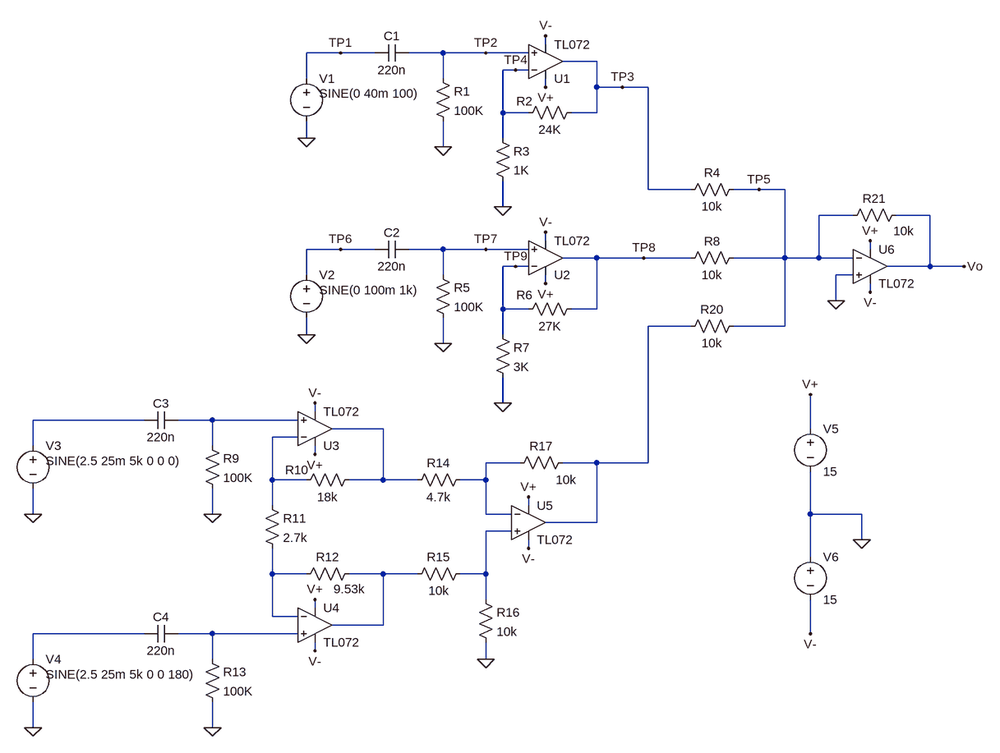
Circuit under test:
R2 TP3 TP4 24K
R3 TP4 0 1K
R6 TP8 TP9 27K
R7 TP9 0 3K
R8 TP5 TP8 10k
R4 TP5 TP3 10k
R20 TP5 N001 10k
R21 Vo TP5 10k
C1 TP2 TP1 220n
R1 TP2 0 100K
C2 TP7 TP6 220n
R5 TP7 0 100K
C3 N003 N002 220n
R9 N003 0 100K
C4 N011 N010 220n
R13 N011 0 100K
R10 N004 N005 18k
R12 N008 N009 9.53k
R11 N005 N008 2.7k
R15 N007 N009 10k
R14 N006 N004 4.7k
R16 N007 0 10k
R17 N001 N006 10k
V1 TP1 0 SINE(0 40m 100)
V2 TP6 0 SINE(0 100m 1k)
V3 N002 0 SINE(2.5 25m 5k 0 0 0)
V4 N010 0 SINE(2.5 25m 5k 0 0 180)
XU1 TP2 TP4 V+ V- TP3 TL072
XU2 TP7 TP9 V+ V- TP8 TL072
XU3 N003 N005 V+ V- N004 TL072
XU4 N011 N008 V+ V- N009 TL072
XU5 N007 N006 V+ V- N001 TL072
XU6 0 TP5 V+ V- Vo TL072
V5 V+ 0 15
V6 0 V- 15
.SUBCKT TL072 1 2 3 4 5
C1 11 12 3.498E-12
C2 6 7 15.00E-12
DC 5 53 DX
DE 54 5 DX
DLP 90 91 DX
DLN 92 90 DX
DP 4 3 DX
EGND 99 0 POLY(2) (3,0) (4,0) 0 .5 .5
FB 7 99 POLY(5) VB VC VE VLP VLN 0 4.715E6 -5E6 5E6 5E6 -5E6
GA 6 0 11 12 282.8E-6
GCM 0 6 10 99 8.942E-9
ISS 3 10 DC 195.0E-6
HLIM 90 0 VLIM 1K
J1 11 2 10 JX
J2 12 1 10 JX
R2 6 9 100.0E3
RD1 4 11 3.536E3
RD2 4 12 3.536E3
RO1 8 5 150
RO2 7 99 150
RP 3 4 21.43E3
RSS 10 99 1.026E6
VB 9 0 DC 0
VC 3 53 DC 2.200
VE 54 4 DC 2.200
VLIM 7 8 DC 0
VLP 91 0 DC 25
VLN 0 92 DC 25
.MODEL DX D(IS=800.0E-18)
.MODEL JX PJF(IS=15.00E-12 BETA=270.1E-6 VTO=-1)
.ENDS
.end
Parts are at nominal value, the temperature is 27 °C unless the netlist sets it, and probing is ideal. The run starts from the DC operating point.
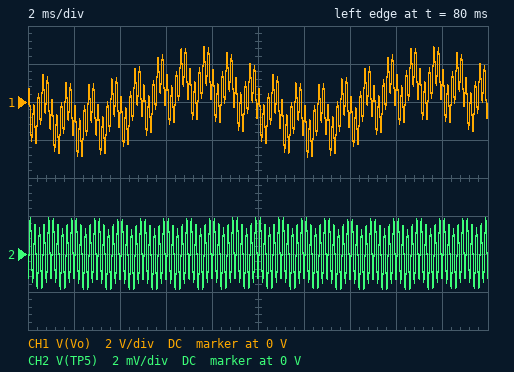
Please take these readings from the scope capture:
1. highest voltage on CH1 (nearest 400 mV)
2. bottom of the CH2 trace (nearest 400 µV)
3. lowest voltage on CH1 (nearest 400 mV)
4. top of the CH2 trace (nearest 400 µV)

2.8 V
-2.0 mV
-2.8 V
2.0 mV
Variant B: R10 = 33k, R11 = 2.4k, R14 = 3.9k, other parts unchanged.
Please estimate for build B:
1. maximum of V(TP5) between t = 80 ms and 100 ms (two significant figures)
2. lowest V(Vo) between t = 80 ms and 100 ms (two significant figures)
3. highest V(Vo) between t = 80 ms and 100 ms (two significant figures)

3.6 mV
-4.0 V
4.0 V
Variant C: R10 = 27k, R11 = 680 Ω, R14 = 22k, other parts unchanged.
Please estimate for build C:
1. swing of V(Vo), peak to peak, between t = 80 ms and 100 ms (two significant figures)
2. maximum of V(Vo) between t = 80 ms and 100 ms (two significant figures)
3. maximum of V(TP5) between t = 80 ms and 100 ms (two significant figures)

6.5 V
3.2 V
2.4 mV
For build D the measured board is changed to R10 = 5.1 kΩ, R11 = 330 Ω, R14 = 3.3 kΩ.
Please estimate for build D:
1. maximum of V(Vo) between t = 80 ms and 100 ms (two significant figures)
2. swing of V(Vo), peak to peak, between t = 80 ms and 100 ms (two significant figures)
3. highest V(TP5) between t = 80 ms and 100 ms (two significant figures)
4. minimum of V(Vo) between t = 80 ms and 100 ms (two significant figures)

7.2 V
14 V
8.2 mV
-7.2 V
